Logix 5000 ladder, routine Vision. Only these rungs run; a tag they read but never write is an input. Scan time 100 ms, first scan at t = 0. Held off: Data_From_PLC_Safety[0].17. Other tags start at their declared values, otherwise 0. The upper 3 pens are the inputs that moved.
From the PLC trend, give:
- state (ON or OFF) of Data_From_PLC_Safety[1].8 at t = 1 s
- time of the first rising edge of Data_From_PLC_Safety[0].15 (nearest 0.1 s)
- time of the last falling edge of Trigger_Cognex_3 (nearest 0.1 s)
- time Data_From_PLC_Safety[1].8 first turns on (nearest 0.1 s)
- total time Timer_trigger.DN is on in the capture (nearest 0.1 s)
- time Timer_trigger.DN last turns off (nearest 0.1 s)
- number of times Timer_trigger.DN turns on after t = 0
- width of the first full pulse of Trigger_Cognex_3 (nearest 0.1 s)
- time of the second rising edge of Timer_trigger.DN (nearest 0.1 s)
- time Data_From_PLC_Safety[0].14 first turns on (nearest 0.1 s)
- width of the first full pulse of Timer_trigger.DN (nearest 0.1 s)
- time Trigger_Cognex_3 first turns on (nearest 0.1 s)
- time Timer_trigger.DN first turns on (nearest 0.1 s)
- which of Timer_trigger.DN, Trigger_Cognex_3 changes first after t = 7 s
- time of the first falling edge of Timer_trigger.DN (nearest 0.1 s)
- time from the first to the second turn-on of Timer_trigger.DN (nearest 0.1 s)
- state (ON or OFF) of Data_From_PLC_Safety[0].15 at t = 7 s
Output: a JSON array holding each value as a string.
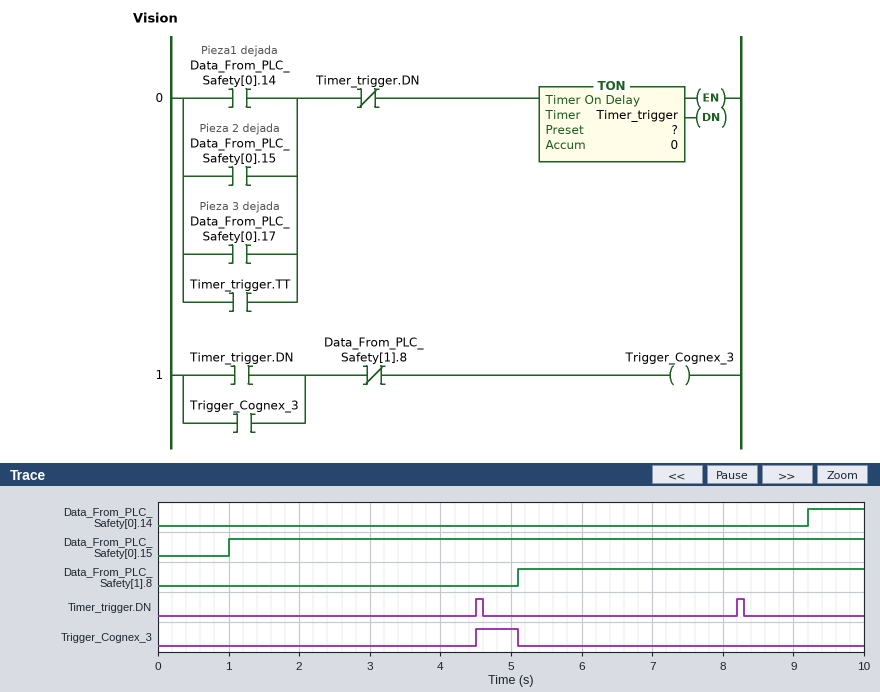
["OFF", "1.0 s", "5.1 s", "5.1 s", "0.2 s", "8.3 s", "2", "0.6 s", "8.2 s", "9.2 s", "0.1 s", "4.5 s", "4.5 s", "Timer_trigger.DN", "4.6 s", "3.7 s", "ON"]
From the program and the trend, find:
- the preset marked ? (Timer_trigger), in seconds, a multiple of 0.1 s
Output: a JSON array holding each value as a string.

["3.5 s"]
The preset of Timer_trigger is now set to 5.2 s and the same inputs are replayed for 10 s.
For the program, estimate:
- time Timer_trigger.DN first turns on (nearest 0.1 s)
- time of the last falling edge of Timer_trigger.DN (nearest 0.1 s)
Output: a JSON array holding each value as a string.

["6.2 s", "6.3 s"]
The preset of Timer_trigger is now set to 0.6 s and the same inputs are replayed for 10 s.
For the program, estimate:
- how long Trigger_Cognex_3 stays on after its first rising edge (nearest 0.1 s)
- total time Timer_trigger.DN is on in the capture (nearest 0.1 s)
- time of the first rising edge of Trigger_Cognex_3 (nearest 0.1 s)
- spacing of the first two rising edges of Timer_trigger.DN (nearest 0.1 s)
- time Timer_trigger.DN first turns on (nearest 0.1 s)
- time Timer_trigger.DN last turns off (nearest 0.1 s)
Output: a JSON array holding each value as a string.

["3.5 s", "1.1 s", "1.6 s", "0.8 s", "1.6 s", "9.7 s"]
